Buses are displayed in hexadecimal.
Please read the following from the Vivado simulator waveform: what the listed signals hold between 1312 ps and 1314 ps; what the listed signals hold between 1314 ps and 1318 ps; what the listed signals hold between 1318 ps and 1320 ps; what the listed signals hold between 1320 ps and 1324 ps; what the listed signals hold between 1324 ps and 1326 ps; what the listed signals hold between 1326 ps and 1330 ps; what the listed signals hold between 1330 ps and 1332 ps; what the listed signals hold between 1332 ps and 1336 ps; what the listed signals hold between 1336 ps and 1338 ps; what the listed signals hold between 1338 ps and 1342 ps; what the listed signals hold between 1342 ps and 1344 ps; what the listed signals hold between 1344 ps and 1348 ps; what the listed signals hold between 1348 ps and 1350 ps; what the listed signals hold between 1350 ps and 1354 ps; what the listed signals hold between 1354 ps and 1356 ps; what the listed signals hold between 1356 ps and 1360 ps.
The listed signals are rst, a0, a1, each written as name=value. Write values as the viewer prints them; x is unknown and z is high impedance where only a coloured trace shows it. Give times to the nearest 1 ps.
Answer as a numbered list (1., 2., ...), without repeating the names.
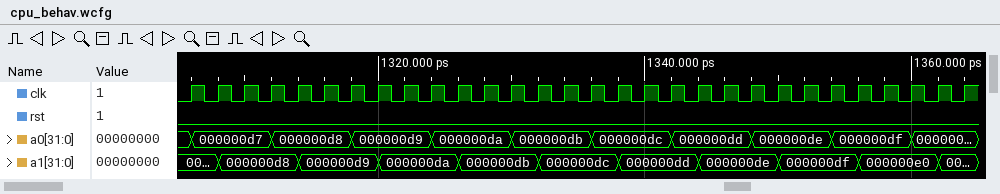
1. rst=0, a0=000000d8, a1=000000d8
2. rst=0, a0=000000d8, a1=000000d9
3. rst=0, a0=000000d9, a1=000000d9
4. rst=0, a0=000000d9, a1=000000da
5. rst=0, a0=000000da, a1=000000da
6. rst=0, a0=000000da, a1=000000db
7. rst=0, a0=000000db, a1=000000db
8. rst=0, a0=000000db, a1=000000dc
9. rst=0, a0=000000dc, a1=000000dc
10. rst=0, a0=000000dc, a1=000000dd
11. rst=0, a0=000000dd, a1=000000dd
12. rst=0, a0=000000dd, a1=000000de
13. rst=0, a0=000000de, a1=000000de
14. rst=0, a0=000000de, a1=000000df
15. rst=0, a0=000000df, a1=000000df
16. rst=0, a0=000000df, a1=000000e0
